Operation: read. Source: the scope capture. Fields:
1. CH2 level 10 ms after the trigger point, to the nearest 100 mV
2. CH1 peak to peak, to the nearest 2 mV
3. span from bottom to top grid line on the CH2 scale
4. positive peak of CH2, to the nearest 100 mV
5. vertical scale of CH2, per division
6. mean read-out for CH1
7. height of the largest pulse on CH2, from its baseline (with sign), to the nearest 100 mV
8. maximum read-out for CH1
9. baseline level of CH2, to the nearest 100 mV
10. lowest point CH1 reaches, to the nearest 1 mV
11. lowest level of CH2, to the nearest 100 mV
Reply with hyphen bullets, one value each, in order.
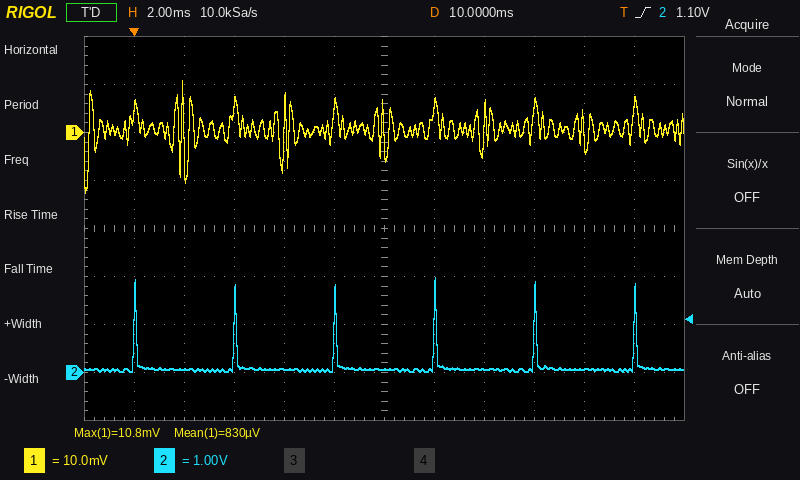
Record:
- 100 mV
- 24 mV
- 8 V
- 2.0 V
- 1 V
- 830 µV
- +1.9 V
- 10.8 mV
- 100 mV
- -12 mV
- 0.0 V
